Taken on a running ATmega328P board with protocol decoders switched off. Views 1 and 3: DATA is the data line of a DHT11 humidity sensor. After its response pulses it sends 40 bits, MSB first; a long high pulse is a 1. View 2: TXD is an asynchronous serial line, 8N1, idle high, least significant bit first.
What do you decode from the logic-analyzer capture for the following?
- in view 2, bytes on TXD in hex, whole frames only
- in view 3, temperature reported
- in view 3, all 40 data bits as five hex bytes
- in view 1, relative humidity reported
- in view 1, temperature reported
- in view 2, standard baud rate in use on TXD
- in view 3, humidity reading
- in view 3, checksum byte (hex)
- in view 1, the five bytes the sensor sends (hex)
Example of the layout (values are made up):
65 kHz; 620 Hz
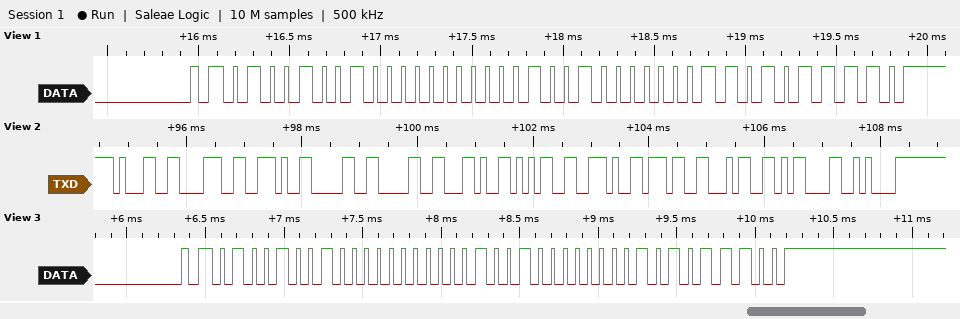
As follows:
31 38 2E 30 30 2C 35 2E 37 34 0D 0A; 18.1 °C; 49 00 12 01 5C; 73 %; 18.3 °C; 9600 baud; 73 %; 0x5C; 49 00 12 03 5E
